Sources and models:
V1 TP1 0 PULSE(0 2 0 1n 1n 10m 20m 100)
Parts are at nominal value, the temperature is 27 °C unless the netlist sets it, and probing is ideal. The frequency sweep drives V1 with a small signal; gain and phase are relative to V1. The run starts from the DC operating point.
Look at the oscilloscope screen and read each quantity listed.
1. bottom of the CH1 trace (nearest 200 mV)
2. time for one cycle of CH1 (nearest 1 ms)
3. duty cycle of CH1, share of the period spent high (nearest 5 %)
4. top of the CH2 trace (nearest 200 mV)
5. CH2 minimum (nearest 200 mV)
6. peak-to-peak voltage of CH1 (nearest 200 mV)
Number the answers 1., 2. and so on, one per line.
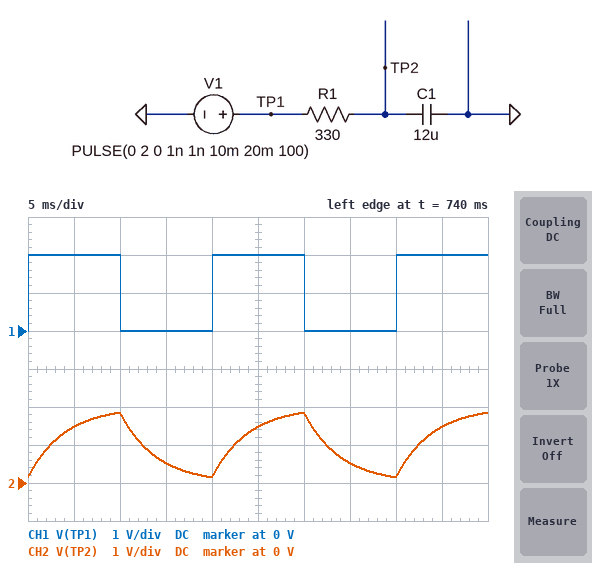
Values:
1. 0 V
2. 20 ms
3. 50 %
4. 1.8 V
5. 200 mV
6. 2.0 V
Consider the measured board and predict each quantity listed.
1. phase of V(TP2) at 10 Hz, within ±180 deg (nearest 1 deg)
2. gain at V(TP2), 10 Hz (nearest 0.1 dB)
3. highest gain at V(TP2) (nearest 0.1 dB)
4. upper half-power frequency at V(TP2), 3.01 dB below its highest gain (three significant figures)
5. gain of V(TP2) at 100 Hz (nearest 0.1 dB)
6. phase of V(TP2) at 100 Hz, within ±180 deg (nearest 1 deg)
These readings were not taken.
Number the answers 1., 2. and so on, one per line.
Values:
1. -14 deg
2. -0.3 dB
3. 0 dB
4. 40.2 Hz
5. -8.6 dB
6. -68 deg
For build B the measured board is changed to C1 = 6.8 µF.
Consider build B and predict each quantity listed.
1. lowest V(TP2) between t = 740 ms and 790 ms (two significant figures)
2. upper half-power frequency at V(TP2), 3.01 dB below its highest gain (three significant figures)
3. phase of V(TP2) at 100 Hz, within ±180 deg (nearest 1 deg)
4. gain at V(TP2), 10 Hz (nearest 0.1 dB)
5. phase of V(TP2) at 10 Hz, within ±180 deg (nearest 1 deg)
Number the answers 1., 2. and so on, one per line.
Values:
1. 23 mV
2. 70.9 Hz
3. -55 deg
4. -0.1 dB
5. -8 deg
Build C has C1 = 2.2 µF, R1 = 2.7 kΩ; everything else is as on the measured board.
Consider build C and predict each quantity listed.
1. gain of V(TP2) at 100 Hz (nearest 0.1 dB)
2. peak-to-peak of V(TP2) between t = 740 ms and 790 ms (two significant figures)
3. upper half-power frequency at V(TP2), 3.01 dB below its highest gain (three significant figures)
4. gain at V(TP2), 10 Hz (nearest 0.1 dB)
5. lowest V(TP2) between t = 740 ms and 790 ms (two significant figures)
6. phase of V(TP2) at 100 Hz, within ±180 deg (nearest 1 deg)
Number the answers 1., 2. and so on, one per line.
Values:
1. -11.7 dB
2. 1.4 V
3. 26.8 Hz
4. -0.6 dB
5. 310 mV
6. -75 deg
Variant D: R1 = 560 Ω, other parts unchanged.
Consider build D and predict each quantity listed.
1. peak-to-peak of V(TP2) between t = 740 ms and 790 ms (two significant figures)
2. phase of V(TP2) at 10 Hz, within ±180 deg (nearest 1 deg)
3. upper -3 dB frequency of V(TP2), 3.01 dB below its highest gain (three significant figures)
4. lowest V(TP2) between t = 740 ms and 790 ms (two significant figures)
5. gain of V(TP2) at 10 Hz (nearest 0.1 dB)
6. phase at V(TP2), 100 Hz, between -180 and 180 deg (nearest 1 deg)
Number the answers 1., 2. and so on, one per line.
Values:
1. 1.3 V
2. -23 deg
3. 23.7 Hz
4. 370 mV
5. -0.7 dB
6. -77 deg
